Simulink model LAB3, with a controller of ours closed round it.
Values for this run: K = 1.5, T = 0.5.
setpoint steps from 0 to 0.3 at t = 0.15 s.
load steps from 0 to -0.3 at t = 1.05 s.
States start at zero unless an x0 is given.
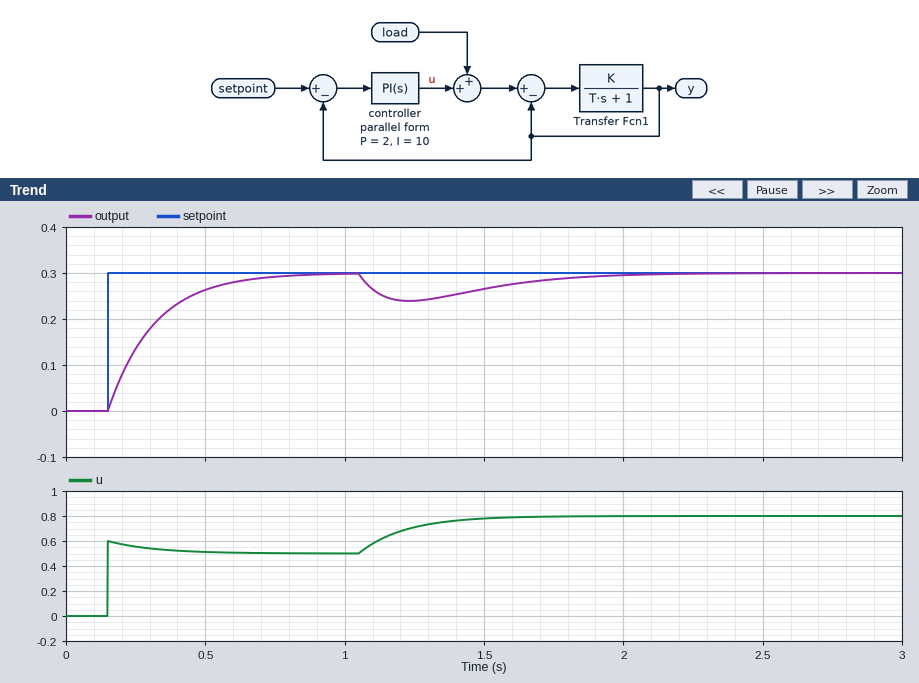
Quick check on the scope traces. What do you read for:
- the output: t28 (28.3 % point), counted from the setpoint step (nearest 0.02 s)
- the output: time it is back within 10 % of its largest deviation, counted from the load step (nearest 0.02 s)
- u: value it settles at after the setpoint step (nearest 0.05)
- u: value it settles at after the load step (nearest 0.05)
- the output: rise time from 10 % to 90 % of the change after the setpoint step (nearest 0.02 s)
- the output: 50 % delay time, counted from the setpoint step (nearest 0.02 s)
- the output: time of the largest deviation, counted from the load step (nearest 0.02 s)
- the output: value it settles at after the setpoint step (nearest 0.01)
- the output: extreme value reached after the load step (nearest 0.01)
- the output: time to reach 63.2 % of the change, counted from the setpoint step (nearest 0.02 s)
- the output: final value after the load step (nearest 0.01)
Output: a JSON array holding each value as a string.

["0.06 s", "0.90 s", "0.50", "0.80", "0.36 s", "0.12 s", "0.18 s", "0.30", "0.24", "0.16 s", "0.30"]
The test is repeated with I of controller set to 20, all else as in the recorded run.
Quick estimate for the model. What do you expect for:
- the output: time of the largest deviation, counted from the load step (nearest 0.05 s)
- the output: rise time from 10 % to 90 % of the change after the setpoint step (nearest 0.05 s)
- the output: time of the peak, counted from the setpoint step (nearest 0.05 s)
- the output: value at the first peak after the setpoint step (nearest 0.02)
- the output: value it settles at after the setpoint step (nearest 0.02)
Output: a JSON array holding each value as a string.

["0.15 s", "0.20 s", "0.40 s", "0.32", "0.30"]
